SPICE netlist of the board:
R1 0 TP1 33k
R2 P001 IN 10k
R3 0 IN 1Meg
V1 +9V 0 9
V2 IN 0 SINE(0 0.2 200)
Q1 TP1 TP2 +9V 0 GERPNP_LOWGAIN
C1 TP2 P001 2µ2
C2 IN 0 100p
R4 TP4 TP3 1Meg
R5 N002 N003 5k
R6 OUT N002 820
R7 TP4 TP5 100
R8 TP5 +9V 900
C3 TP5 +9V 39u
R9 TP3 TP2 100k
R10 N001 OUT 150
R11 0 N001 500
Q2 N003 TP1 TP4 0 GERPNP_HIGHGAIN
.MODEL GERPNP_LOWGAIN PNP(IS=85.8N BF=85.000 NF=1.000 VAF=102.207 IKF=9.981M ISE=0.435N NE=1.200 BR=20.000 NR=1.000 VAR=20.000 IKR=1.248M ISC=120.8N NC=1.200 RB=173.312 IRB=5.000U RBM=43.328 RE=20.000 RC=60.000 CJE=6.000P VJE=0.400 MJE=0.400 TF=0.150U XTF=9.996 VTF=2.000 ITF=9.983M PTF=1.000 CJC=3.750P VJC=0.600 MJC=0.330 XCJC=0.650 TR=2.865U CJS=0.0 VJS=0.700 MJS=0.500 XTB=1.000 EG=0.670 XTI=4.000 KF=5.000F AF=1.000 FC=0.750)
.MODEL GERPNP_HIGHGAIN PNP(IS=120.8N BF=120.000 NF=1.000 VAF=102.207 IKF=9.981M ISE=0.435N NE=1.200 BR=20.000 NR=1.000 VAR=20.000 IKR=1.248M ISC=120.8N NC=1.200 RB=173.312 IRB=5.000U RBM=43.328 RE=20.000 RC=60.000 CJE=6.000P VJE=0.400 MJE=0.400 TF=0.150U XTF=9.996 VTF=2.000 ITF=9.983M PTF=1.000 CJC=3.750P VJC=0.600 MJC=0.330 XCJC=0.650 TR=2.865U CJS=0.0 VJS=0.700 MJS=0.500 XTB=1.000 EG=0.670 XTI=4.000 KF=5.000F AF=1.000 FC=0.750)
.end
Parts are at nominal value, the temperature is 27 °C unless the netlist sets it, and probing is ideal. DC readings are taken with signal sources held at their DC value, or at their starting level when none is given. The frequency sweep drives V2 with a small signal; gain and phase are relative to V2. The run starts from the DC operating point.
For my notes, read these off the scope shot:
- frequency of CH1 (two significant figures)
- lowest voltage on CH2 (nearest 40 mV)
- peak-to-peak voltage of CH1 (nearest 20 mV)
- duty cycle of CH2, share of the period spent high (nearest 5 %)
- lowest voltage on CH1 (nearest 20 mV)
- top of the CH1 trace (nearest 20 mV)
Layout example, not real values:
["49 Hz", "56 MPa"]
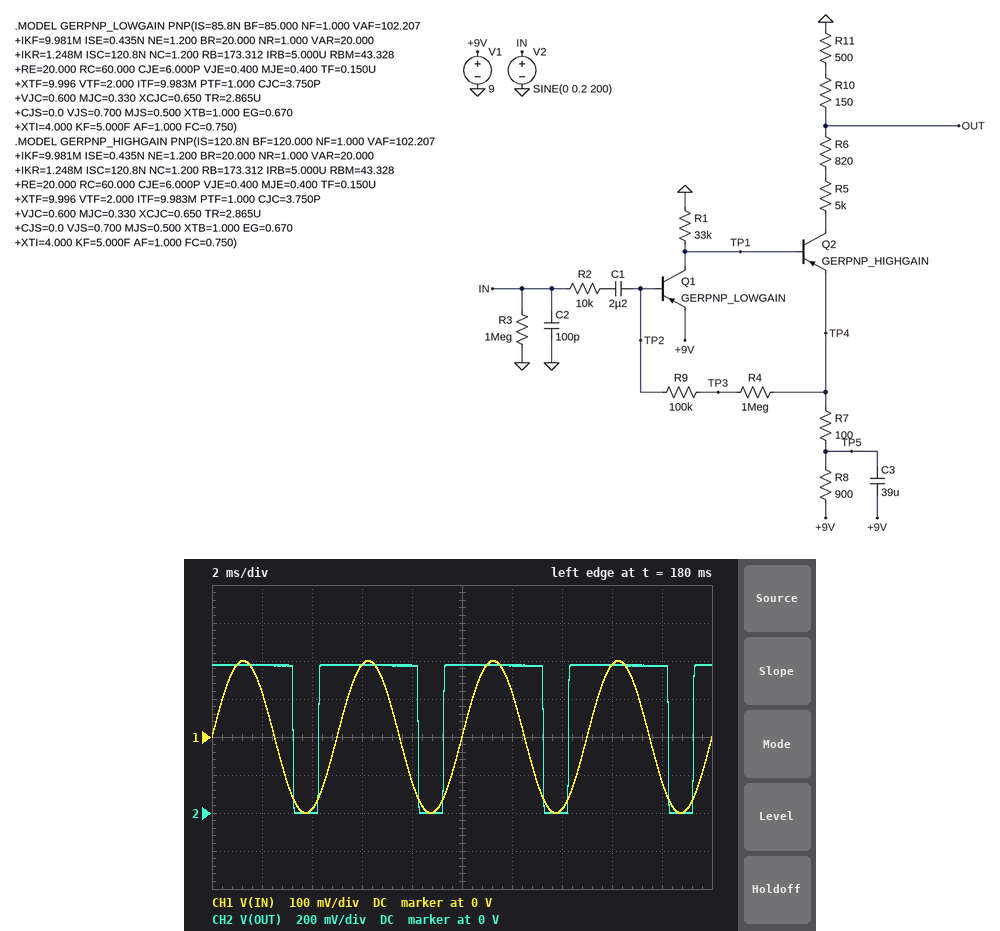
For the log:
["200 Hz", "0 V", "400 mV", "80 %", "-200 mV", "200 mV"]
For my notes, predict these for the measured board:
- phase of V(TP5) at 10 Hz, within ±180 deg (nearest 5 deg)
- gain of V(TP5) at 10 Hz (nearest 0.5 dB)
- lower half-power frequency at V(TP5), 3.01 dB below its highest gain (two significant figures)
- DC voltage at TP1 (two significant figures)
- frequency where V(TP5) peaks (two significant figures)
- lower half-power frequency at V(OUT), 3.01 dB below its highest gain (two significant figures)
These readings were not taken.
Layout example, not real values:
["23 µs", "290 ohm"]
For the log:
["130 deg", "-2.5 dB", "1.3 Hz", "7.4 V", "3.4 Hz", "1.3 Hz"]
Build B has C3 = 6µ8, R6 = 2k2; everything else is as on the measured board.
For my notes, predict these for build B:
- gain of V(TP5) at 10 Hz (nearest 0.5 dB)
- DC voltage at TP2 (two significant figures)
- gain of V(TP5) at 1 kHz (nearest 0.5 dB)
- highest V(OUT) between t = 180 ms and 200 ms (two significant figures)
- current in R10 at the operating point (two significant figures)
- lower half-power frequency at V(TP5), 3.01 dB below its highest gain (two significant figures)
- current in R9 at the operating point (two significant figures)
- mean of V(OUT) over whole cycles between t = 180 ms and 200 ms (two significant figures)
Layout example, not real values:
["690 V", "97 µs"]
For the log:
["3.0 dB", "8.8 V", "-27.0 dB", "660 mV", "990 µA", "1.8 Hz", "880 nA", "530 mV"]
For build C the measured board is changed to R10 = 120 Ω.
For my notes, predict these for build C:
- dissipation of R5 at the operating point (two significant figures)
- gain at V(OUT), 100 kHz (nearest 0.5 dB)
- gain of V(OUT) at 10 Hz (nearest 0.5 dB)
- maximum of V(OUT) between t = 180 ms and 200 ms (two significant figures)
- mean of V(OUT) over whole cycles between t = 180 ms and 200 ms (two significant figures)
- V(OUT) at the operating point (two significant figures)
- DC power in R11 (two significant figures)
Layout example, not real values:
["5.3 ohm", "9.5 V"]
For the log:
["6.9 mW", "-38.5 dB", "-23.5 dB", "750 mV", "590 mV", "730 mV", "690 µW"]
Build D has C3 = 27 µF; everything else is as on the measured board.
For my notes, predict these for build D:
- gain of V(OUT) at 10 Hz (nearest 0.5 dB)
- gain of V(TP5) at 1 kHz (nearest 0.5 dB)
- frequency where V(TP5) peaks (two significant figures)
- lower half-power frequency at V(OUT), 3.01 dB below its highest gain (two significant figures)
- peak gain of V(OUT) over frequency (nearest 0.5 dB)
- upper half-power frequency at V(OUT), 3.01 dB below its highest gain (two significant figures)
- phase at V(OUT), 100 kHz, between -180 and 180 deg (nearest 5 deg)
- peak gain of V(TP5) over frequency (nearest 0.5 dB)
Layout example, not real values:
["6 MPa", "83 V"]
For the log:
["-20.5 dB", "-38.0 dB", "4.1 Hz", "1.5 Hz", "-18.5 dB", "11 Hz", "125 deg", "2.0 dB"]
